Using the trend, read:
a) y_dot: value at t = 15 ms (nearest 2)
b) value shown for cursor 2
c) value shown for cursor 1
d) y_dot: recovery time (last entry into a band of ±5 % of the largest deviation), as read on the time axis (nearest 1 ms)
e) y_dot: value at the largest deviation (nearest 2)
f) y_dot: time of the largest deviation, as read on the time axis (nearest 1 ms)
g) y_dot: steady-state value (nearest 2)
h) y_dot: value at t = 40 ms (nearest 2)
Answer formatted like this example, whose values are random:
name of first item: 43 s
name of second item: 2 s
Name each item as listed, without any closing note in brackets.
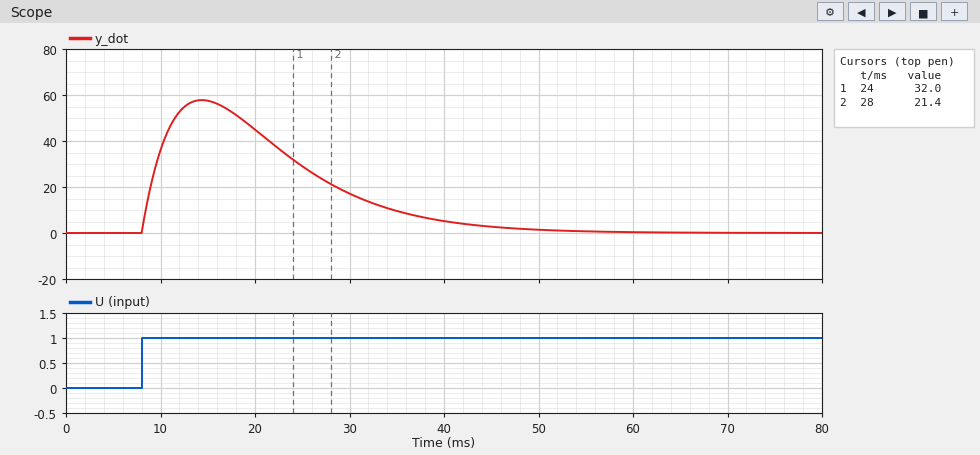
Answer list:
y_dot: value at t = 15 ms: 58
value shown for cursor 2: 21.4
value shown for cursor 1: 32.0
y_dot: recovery time (last entry into a band of ±5 % of the largest deviation), as read on the time axis: 45 ms
y_dot: value at the largest deviation: 58
y_dot: time of the largest deviation, as read on the time axis: 14 ms
y_dot: steady-state value: 0
y_dot: value at t = 40 ms: 6
